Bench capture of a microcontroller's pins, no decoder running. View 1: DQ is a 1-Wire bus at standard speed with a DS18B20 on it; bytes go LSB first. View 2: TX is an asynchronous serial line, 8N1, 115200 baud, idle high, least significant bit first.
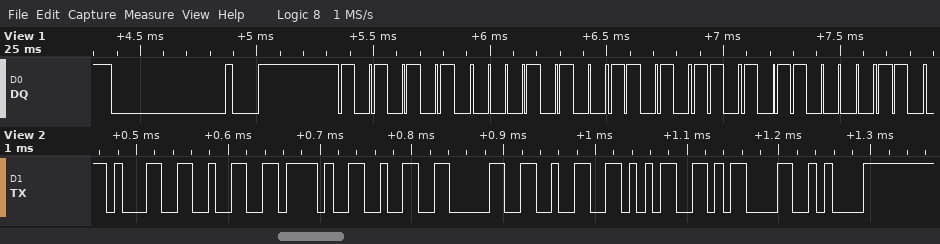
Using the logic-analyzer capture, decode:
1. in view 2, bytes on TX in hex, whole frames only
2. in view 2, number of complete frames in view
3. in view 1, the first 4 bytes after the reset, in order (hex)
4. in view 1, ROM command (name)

31 32 2F 32 30 32 35 0D 0A
9
55 28 6B 0D
Match ROM
